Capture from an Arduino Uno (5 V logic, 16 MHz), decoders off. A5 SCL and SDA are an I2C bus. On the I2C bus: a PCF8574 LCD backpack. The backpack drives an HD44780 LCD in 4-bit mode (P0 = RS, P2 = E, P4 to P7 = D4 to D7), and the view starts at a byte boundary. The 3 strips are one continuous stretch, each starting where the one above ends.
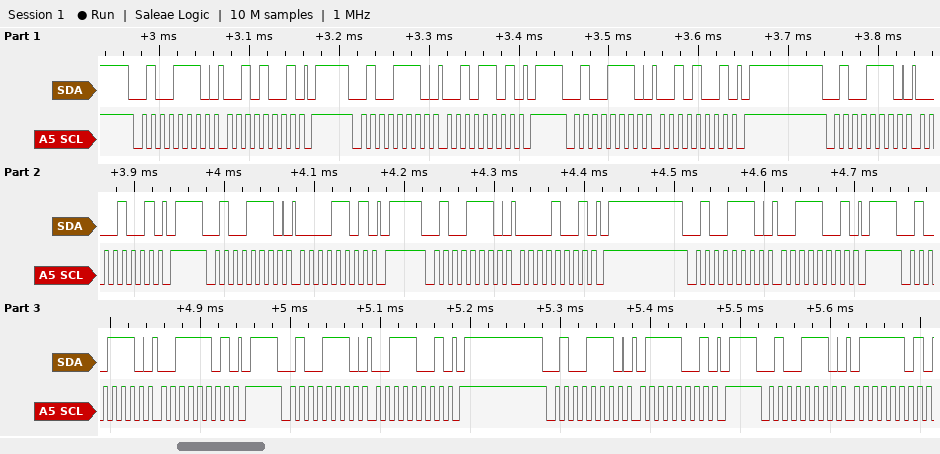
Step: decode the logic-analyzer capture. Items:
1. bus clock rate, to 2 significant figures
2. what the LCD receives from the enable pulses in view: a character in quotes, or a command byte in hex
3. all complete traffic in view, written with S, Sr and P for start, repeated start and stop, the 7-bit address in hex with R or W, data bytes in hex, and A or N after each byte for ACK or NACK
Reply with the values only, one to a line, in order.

100 kHz
' '
S 27W A 29 A P S 27W A 2D A P S 27W A 29 A P S 27W A 09 A P S 27W A 0D A P S 27W A 09 A P S 27W A 39 A P S 27W A 3D A P S 27W A 39 A P S 27W A 79 A P S 27W A 7D A
